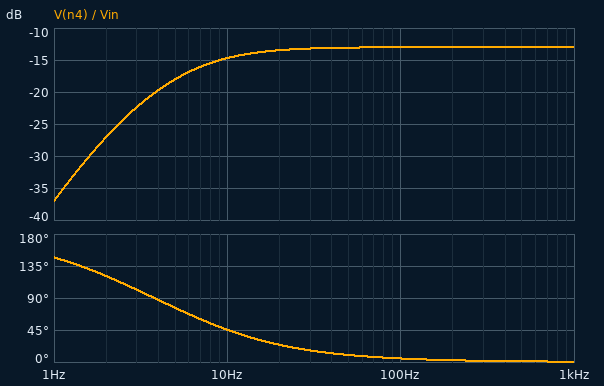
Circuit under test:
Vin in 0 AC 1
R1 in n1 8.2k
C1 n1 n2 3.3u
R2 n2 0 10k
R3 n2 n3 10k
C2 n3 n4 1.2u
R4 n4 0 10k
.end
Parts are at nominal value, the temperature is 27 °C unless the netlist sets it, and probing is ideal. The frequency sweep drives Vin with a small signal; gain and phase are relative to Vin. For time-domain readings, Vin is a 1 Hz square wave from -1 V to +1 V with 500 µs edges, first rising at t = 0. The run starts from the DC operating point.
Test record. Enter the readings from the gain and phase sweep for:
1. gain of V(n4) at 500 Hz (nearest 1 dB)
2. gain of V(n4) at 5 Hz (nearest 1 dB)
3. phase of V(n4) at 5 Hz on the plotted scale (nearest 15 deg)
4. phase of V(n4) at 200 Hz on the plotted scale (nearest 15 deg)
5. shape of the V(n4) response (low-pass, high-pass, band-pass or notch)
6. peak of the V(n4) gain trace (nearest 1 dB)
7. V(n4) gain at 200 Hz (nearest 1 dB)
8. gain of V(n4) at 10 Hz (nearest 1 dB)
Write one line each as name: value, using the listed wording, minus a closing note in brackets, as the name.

gain of V(n4) at 500 Hz: -13 dB
gain of V(n4) at 5 Hz: -18 dB
phase of V(n4) at 5 Hz on the plotted scale: 75 deg
phase of V(n4) at 200 Hz on the plotted scale: 0 deg
shape of the V(n4) response: high-pass
peak of the V(n4) gain trace: -13 dB
V(n4) gain at 200 Hz: -13 dB
gain of V(n4) at 10 Hz: -15 dB
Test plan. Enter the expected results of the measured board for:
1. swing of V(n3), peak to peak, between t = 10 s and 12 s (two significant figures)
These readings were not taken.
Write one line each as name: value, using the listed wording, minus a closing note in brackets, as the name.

swing of V(n3), peak to peak, between t = 10 s and 12 s: 1.1 V
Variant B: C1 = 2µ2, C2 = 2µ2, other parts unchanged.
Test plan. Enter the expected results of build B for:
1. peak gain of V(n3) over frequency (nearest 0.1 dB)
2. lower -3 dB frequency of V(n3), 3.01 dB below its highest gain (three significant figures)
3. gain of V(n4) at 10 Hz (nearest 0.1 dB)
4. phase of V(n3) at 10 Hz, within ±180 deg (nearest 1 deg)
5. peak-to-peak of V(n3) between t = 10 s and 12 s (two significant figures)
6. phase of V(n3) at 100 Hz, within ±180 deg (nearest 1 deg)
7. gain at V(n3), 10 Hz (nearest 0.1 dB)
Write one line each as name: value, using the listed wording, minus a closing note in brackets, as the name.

peak gain of V(n3) over frequency: -12.4 dB
lower -3 dB frequency of V(n3), 3.01 dB below its highest gain: 1.57 Hz
gain of V(n4) at 10 Hz: -14.4 dB
phase of V(n3) at 10 Hz, within ±180 deg: 6 deg
peak-to-peak of V(n3) between t = 10 s and 12 s: 890 mV
phase of V(n3) at 100 Hz, within ±180 deg: 0 deg
gain at V(n3), 10 Hz: -12.6 dB
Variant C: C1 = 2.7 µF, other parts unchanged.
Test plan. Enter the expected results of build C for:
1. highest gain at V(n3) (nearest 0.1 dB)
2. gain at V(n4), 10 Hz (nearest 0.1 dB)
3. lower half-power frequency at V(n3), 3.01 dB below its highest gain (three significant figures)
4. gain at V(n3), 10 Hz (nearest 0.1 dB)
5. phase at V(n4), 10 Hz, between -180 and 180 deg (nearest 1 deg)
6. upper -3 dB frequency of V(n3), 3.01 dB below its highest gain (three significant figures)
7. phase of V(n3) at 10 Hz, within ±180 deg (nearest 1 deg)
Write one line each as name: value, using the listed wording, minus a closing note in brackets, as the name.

highest gain at V(n3): -9.5 dB
gain at V(n4), 10 Hz: -14.9 dB
lower half-power frequency at V(n3), 3.01 dB below its highest gain: 1.71 Hz
gain at V(n3), 10 Hz: -10.5 dB
phase at V(n4), 10 Hz, between -180 and 180 deg: 49 deg
upper -3 dB frequency of V(n3), 3.01 dB below its highest gain: 31.9 Hz
phase of V(n3) at 10 Hz, within ±180 deg: -4 deg
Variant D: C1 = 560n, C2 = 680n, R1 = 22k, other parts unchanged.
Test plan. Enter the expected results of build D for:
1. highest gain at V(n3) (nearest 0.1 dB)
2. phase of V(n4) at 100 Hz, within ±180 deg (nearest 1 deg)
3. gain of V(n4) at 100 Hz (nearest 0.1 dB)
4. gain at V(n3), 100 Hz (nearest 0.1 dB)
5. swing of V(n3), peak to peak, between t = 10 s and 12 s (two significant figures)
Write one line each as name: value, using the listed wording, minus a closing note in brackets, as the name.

highest gain at V(n3): -16.0 dB
phase of V(n4) at 100 Hz, within ±180 deg: 11 deg
gain of V(n4) at 100 Hz: -18.8 dB
gain at V(n3), 100 Hz: -18.5 dB
swing of V(n3), peak to peak, between t = 10 s and 12 s: 500 mV
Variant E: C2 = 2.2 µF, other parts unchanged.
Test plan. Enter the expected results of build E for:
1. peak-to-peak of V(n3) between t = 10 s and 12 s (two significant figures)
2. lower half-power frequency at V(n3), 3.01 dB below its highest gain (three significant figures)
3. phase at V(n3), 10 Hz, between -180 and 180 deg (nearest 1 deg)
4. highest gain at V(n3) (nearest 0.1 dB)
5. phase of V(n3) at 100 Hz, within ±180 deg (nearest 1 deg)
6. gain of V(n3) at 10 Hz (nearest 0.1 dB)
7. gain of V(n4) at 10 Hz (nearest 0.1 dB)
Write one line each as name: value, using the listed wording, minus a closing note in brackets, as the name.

peak-to-peak of V(n3) between t = 10 s and 12 s: 930 mV
lower half-power frequency at V(n3), 3.01 dB below its highest gain: 1.20 Hz
phase at V(n3), 10 Hz, between -180 and 180 deg: -2 deg
highest gain at V(n3): -10.9 dB
phase of V(n3) at 100 Hz, within ±180 deg: -1 deg
gain of V(n3) at 10 Hz: -12.1 dB
gain of V(n4) at 10 Hz: -13.9 dB
